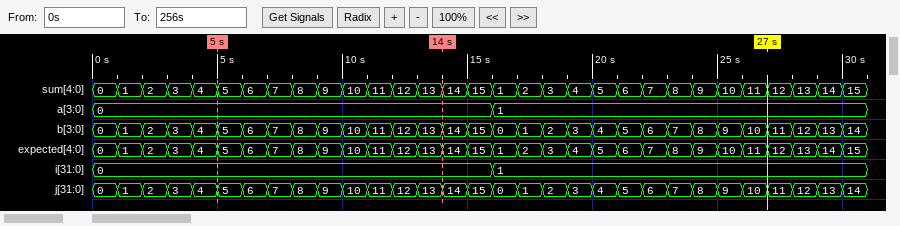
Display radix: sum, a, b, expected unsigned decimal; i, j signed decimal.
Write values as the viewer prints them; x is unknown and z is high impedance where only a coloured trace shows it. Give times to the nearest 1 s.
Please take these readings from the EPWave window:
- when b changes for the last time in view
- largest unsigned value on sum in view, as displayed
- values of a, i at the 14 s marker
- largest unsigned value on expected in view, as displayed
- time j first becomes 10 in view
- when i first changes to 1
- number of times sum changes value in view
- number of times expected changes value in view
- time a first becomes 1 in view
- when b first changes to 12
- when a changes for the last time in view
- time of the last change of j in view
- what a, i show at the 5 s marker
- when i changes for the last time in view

30 s
15
a=0, i=0
15
10 s
16 s
30
30
16 s
12 s
16 s
30 s
a=0, i=0
16 s
